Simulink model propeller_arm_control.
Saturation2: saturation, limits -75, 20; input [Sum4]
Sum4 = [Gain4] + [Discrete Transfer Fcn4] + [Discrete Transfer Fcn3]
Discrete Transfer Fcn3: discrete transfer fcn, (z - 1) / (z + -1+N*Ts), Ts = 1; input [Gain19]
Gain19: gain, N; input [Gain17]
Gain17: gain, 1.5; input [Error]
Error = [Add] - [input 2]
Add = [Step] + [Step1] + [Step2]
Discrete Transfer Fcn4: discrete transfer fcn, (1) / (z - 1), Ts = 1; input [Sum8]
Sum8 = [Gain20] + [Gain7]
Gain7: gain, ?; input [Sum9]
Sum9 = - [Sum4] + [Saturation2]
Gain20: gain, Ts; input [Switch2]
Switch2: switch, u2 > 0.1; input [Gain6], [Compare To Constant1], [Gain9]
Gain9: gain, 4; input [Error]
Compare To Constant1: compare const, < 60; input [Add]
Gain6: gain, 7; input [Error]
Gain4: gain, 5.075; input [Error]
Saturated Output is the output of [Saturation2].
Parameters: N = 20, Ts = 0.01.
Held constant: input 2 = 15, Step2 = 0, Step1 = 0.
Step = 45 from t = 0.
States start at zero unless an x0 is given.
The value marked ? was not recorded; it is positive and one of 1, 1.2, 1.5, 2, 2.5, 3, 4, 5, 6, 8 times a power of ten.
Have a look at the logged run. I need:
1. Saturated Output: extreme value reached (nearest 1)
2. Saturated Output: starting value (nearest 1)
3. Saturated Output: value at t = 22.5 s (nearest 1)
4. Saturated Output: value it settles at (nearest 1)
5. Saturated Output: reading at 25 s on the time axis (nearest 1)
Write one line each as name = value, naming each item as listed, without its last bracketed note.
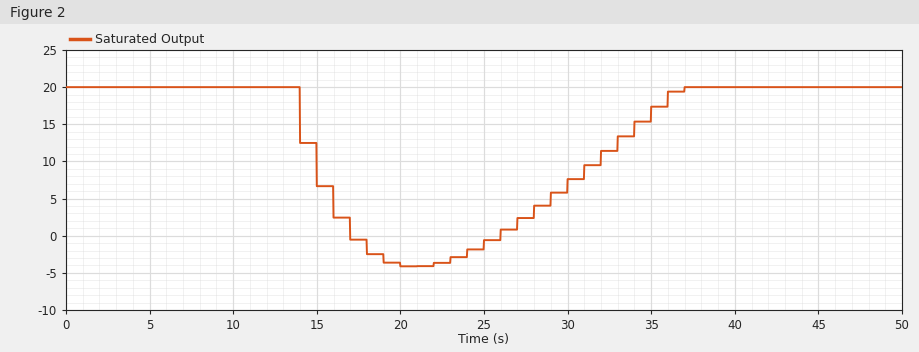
Saturated Output: extreme value reached = -4
Saturated Output: starting value = 20
Saturated Output: value at t = 22.5 s = -4
Saturated Output: value it settles at = 20
Saturated Output: reading at 25 s on the time axis = -1
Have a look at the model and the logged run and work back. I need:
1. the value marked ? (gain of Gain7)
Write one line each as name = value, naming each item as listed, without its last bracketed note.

the value marked ? = 0.05
